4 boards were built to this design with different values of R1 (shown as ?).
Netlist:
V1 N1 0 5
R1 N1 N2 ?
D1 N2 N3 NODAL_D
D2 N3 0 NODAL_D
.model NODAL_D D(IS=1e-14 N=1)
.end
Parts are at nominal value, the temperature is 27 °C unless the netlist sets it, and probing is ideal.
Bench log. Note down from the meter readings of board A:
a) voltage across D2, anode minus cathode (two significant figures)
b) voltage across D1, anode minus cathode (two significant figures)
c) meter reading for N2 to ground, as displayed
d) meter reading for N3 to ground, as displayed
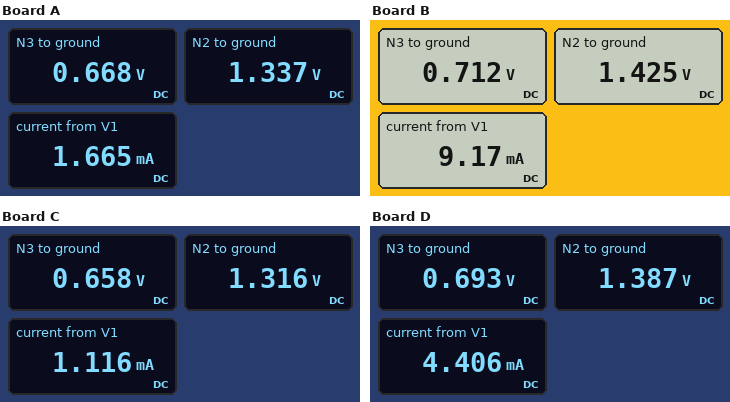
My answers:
670 mV
670 mV
1.337 V
0.668 V
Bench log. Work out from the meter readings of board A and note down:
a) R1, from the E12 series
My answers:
2.2 kΩ
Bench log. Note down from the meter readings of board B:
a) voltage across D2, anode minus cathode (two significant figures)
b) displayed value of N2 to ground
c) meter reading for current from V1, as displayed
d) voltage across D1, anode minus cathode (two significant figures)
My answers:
710 mV
1.425 V
9.17 mA
710 mV
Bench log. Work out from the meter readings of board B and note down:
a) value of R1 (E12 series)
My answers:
390 Ω
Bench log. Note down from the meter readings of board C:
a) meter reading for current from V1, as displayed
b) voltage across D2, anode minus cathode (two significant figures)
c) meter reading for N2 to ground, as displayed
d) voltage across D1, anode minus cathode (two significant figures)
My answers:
1.116 mA
660 mV
1.316 V
660 mV
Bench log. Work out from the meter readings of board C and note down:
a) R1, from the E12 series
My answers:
3.3 kΩ
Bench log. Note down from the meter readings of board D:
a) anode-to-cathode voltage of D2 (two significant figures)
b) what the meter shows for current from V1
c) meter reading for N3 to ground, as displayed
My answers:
690 mV
4.406 mA
0.693 V
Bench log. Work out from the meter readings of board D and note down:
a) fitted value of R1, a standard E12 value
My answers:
820 Ω
